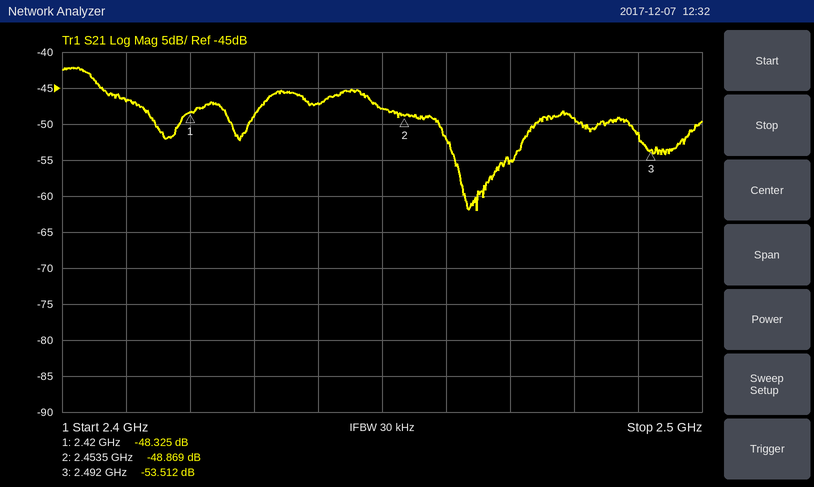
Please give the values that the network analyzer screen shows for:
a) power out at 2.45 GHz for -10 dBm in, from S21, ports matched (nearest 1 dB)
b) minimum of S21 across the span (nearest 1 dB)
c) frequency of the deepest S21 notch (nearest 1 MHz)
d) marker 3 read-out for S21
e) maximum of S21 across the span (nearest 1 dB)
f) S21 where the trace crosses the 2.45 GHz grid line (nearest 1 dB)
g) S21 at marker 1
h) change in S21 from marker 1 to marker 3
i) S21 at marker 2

-58 dBm
-62 dB
2.465 GHz
-53.512 dB
-42 dB
-48 dB
-48.325 dB
-5.187 dB
-48.869 dB
